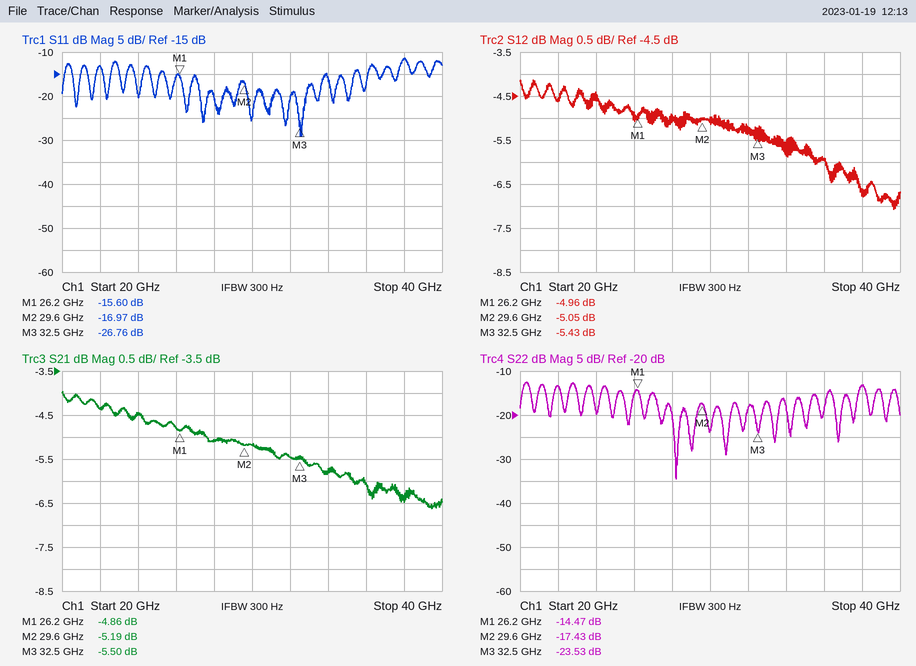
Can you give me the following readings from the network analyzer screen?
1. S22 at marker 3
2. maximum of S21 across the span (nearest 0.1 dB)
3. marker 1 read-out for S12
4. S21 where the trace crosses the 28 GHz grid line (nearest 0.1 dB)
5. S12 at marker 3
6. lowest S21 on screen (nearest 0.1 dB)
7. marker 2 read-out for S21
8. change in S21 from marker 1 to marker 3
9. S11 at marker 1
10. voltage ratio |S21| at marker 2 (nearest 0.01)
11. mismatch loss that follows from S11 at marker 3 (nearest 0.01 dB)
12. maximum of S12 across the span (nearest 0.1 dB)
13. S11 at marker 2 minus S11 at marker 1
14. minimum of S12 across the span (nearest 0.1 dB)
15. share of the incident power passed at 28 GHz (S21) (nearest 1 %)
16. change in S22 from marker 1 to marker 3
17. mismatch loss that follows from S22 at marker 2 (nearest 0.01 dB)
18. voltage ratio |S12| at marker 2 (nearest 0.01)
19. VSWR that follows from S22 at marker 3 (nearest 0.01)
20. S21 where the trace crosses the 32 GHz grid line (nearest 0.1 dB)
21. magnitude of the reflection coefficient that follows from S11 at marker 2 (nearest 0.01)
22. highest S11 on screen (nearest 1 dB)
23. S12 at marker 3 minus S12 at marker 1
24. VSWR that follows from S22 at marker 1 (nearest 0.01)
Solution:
-23.53 dB
-4.0 dB
-4.96 dB
-5.1 dB
-5.43 dB
-6.6 dB
-5.19 dB
-0.64 dB
-15.60 dB
0.55
0.01 dB
-4.1 dB
-1.37 dB
-7.1 dB
31 %
-9.06 dB
0.08 dB
0.56
1.14
-5.5 dB
0.14
-11 dB
-0.47 dB
1.47
